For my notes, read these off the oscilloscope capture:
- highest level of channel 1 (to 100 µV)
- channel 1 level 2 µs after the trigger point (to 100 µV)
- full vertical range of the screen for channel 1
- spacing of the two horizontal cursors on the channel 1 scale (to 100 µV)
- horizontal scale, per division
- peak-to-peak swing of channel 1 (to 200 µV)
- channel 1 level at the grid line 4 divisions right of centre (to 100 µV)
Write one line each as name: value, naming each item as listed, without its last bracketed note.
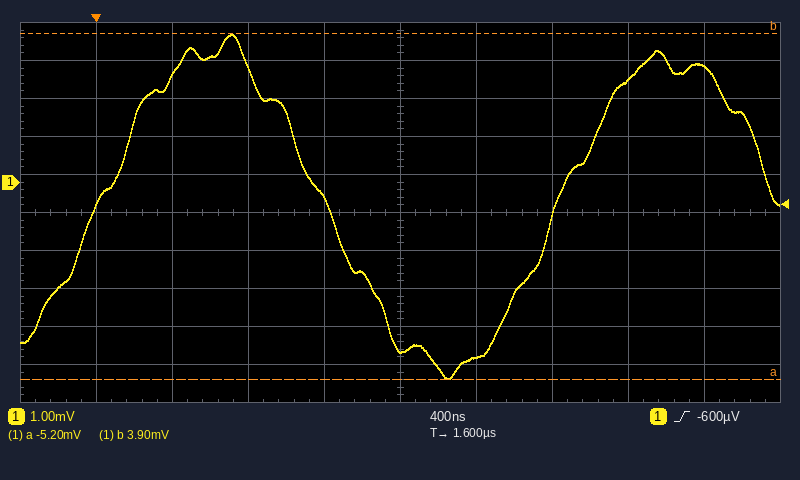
highest level of channel 1: 3.9 mV
channel 1 level 2 µs after the trigger point: -4.6 mV
full vertical range of the screen for channel 1: 10 mV
spacing of the two horizontal cursors on the channel 1 scale: 9.1 mV
horizontal scale, per division: 400 ns
peak-to-peak swing of channel 1: 9.0 mV
channel 1 level at the grid line 4 divisions right of centre: 3.0 mV
